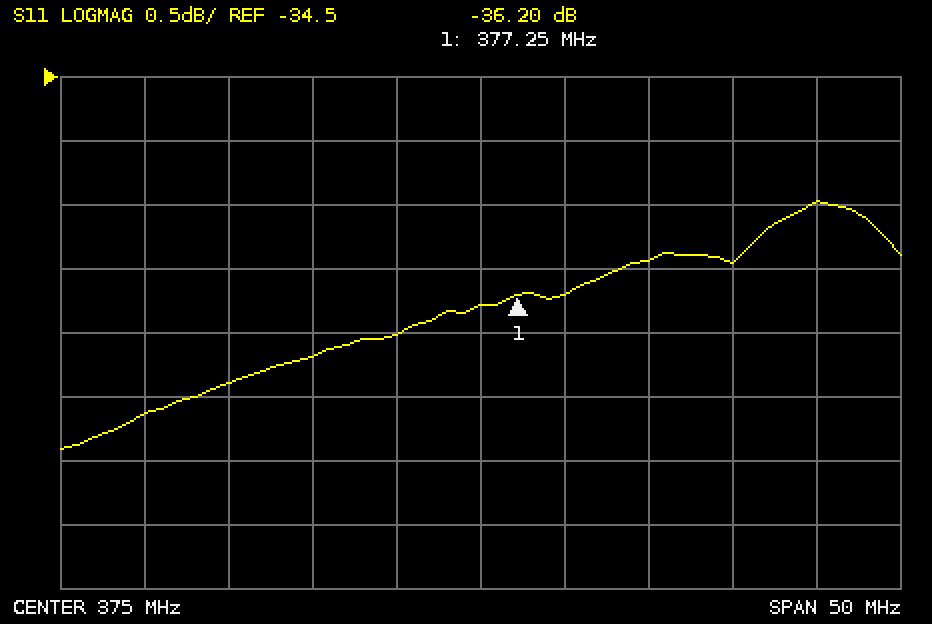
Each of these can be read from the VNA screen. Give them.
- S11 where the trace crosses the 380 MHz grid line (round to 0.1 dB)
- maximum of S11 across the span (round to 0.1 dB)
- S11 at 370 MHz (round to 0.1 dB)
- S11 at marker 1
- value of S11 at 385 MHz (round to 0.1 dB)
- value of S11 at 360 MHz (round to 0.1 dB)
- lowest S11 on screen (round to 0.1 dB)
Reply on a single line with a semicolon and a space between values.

-36.2 dB; -35.5 dB; -36.5 dB; -36.20 dB; -35.9 dB; -36.9 dB; -37.4 dB
